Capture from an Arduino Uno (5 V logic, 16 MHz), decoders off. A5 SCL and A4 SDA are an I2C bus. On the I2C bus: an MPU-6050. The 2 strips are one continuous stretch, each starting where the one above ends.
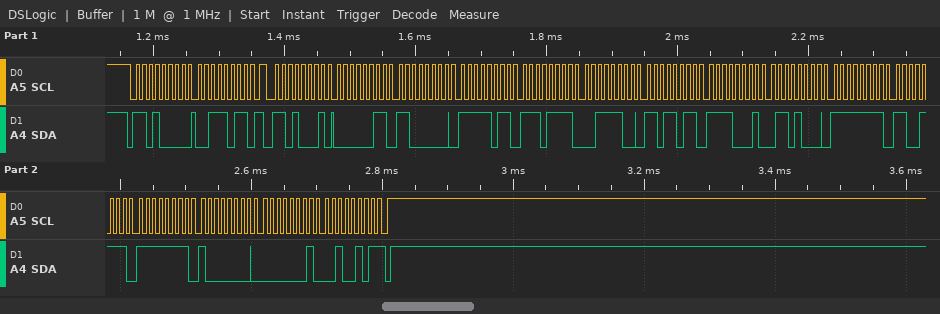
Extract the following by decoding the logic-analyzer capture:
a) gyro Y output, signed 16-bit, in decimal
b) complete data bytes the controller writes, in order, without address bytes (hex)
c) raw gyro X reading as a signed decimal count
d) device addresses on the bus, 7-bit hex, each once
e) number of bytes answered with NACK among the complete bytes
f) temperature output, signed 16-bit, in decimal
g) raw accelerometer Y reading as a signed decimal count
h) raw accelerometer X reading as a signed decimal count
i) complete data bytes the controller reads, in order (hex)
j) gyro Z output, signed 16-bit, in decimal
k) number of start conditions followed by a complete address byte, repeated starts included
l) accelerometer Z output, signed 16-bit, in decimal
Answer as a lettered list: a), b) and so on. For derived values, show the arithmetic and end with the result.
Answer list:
a) 0xFF80 = -128
b) 3B
c) 0xFFCF = -49
d) 0x68
e) 1
f) 0xF168 = -3736
g) 0xFBEF = -1041
h) 0x03C0 = 960
i) 03 C0 FB EF 3C DB F1 68 FF CF FF 80 01 25
j) 0x0125 = 293
k) 2
l) 0x3CDB = 15579
